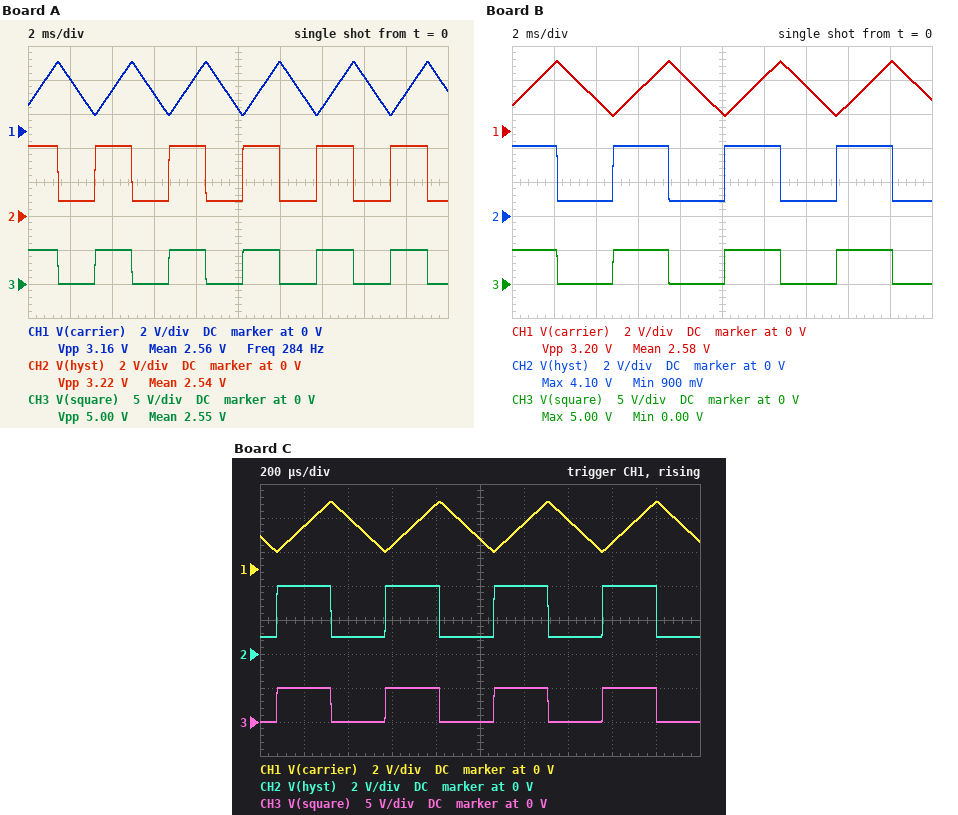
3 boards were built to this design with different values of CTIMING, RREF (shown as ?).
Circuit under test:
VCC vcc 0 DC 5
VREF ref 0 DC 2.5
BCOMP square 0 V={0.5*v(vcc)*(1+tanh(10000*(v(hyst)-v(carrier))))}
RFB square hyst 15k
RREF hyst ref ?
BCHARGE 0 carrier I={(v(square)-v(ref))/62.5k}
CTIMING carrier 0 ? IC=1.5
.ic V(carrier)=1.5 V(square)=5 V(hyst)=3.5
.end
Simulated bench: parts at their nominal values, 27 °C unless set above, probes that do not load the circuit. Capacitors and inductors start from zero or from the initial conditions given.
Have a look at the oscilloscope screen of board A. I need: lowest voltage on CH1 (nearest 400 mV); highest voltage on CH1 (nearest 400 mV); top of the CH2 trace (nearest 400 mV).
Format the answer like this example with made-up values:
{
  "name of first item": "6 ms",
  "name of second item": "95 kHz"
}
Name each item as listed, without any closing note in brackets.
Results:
{
  "lowest voltage on CH1": "800 mV",
  "highest voltage on CH1": "4.0 V",
  "top of the CH2 trace": "4.0 V"
}
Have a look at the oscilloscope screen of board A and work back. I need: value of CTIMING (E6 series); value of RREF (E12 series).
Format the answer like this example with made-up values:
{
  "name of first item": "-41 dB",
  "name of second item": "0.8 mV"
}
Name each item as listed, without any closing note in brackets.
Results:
{
  "value of CTIMING": "22 nF",
  "value of RREF": "27 kΩ"
}
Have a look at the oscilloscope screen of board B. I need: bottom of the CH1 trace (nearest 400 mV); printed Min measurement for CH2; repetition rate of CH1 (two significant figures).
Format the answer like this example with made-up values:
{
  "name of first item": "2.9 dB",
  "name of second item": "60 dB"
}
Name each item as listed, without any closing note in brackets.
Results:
{
  "bottom of the CH1 trace": "800 mV",
  "printed Min measurement for CH2": "900 mV",
  "repetition rate of CH1": "190 Hz"
}
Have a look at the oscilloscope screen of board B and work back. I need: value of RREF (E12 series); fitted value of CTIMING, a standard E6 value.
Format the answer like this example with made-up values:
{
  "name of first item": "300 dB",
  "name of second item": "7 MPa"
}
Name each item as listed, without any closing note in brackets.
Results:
{
  "value of RREF": "27 kΩ",
  "fitted value of CTIMING, a standard E6 value": "33 nF"
}
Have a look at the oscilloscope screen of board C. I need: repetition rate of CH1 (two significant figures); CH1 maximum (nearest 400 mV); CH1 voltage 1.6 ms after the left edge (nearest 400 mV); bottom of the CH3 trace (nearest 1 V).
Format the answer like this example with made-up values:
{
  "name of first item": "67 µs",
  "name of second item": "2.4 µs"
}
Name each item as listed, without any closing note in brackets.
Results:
{
  "repetition rate of CH1": "2.0 kHz",
  "CH1 maximum": "4.0 V",
  "CH1 voltage 1.6 ms after the left edge": "1.6 V",
  "bottom of the CH3 trace": "0 V"
}
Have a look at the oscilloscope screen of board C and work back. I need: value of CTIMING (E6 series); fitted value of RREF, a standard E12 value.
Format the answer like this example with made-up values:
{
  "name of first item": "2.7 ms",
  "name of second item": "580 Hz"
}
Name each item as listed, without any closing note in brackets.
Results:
{
  "value of CTIMING": "3.3 nF",
  "fitted value of RREF, a standard E12 value": "22 kΩ"
}
